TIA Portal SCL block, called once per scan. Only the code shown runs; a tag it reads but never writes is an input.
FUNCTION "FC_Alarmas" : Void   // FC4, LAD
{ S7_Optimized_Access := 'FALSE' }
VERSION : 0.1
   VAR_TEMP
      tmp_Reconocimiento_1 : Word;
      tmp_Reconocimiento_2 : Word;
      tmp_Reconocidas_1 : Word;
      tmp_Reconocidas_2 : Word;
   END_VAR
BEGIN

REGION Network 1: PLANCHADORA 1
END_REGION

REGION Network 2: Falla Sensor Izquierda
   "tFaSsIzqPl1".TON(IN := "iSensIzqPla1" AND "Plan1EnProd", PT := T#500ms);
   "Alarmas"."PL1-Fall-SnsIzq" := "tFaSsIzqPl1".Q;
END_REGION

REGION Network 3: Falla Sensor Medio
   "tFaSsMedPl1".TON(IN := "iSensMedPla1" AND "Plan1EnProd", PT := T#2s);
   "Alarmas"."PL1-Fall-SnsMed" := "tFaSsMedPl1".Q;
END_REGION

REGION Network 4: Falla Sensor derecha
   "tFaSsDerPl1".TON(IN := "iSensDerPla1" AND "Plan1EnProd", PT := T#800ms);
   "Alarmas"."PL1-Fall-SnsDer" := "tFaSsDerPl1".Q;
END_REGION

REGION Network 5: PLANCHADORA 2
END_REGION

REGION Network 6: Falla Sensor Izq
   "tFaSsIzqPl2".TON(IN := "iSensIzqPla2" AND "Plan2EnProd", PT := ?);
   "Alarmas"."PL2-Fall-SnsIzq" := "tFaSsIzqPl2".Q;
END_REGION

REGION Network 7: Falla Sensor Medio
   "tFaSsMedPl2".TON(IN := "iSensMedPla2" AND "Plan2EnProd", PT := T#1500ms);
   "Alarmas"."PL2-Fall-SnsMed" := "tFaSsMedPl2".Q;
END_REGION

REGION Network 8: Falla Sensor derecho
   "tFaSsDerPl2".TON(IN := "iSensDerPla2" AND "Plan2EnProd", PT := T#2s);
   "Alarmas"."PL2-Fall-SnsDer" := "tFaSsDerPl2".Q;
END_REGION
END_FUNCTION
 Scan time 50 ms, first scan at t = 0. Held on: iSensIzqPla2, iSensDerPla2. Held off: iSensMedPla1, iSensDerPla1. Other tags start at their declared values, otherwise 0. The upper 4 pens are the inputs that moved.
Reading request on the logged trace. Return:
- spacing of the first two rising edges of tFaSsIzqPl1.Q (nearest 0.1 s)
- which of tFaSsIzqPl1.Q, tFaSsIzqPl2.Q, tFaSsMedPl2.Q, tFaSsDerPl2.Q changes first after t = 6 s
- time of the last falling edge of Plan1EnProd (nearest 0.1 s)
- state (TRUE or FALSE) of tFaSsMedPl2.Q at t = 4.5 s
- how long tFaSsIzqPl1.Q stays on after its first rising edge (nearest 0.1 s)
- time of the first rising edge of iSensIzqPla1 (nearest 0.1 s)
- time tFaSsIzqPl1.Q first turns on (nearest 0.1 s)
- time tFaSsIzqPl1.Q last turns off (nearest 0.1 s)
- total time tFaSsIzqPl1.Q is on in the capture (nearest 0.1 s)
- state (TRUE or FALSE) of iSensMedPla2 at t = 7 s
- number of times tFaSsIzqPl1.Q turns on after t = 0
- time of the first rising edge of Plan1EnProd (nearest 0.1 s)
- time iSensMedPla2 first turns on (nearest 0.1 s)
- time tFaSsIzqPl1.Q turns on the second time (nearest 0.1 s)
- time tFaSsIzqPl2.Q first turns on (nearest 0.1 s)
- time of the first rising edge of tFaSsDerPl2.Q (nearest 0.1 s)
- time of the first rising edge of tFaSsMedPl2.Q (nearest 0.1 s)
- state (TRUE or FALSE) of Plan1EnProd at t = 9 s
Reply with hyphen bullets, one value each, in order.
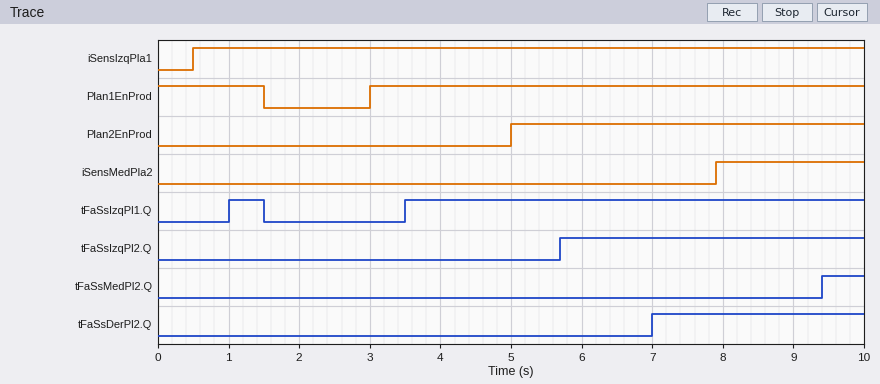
- 2.5 s
- tFaSsDerPl2.Q
- 1.5 s
- FALSE
- 0.5 s
- 0.5 s
- 1.0 s
- 1.5 s
- 7.0 s
- FALSE
- 2
- 3.0 s
- 7.9 s
- 3.5 s
- 5.7 s
- 7.0 s
- 9.4 s
- TRUE
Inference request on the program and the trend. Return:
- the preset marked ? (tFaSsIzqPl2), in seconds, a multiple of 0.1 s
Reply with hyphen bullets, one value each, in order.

- 0.7 s
